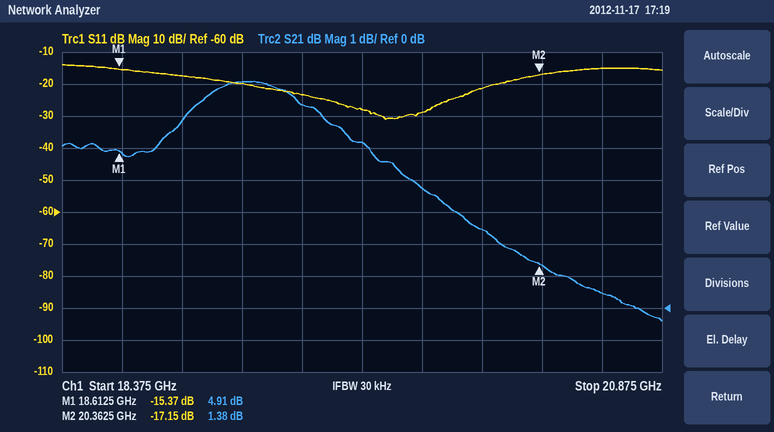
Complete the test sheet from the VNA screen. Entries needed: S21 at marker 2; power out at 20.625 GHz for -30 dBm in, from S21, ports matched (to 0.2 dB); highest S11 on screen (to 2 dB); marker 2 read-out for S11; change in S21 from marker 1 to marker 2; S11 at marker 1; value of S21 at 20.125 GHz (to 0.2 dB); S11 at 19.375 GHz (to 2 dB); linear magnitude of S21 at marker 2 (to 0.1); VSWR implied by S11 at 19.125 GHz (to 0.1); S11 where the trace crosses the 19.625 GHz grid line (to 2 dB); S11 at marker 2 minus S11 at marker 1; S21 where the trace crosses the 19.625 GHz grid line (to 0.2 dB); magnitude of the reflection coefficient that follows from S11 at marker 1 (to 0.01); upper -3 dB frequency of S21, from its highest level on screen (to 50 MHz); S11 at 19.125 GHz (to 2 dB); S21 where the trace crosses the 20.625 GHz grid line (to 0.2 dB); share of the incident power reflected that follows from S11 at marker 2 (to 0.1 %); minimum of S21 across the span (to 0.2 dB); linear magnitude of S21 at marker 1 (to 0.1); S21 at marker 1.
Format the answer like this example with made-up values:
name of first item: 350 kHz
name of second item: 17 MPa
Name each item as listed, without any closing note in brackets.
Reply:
S21 at marker 2: 1.38 dB
power out at 20.625 GHz for -30 dBm in, from S21, ports matched: -29.6 dBm
highest S11 on screen: -14 dB
marker 2 read-out for S11: -17.15 dB
change in S21 from marker 1 to marker 2: -3.53 dB
S11 at marker 1: -15.37 dB
value of S21 at 20.125 GHz: 2.4 dB
S11 at 19.375 GHz: -24 dB
linear magnitude of S21 at marker 2: 1.2
VSWR implied by S11 at 19.125 GHz: 1.2
S11 where the trace crosses the 19.625 GHz grid line: -28 dB
S11 at marker 2 minus S11 at marker 1: -1.78 dB
S21 where the trace crosses the 19.625 GHz grid line: 5.2 dB
magnitude of the reflection coefficient that follows from S11 at marker 1: 0.17
upper -3 dB frequency of S21, from its highest level on screen: 19.80 GHz
S11 at 19.125 GHz: -20 dB
S21 where the trace crosses the 20.625 GHz grid line: 0.4 dB
share of the incident power reflected that follows from S11 at marker 2: 1.9 %
minimum of S21 across the span: -0.4 dB
linear magnitude of S21 at marker 1: 1.8
S21 at marker 1: 4.91 dB
